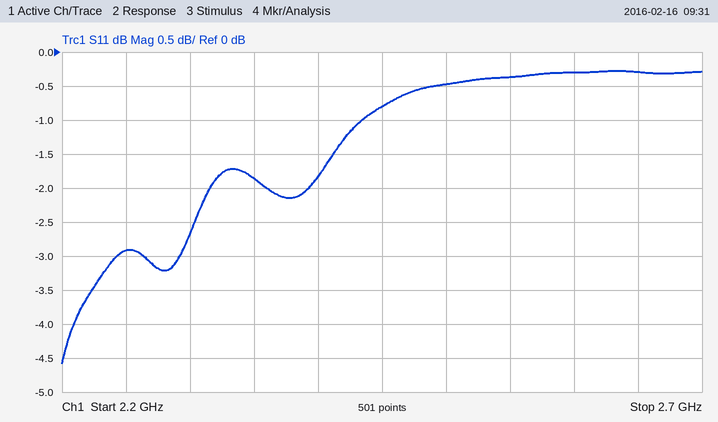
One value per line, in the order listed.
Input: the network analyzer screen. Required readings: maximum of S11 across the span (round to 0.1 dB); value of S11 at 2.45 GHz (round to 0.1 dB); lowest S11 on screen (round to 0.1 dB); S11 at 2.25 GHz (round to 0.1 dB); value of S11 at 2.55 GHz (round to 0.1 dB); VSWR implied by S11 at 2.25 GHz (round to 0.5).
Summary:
-0.3 dB
-0.8 dB
-4.6 dB
-2.9 dB
-0.4 dB
6.0
